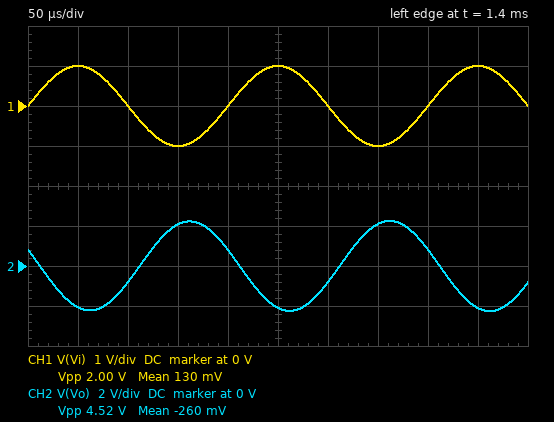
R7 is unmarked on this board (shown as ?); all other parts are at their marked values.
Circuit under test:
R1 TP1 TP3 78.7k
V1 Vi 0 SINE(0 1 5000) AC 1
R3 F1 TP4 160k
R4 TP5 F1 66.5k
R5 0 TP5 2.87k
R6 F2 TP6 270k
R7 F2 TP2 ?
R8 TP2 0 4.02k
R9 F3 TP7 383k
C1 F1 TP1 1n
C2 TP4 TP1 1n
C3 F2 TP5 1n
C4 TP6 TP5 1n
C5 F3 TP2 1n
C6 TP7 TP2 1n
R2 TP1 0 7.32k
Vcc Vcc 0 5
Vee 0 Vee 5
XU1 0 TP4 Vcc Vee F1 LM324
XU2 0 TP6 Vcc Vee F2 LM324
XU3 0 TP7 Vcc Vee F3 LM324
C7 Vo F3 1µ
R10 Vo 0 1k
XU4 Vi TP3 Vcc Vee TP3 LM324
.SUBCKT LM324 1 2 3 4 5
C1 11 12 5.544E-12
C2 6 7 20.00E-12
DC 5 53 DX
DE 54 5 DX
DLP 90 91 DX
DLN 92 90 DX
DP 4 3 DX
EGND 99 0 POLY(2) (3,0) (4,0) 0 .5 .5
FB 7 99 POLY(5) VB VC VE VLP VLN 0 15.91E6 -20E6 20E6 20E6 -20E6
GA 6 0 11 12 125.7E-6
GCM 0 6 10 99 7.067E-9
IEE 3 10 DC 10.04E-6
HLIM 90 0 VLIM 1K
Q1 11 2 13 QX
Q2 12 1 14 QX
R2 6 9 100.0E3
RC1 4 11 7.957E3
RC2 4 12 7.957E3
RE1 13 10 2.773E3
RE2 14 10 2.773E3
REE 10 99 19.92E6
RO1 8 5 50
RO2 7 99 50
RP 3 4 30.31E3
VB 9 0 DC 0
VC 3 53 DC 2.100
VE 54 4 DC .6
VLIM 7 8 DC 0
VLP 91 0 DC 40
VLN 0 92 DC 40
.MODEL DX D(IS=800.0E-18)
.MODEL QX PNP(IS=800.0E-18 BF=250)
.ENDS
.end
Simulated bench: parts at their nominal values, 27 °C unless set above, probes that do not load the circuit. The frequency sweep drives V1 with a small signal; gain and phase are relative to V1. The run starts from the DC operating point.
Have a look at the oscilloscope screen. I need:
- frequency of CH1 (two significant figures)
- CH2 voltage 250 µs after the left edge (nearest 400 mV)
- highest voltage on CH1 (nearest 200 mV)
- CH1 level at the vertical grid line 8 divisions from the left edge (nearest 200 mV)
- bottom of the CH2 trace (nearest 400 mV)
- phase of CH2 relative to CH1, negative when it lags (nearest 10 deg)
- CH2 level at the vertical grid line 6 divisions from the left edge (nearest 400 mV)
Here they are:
5.0 kHz
-2.0 V
1.0 V
0 V
-2.4 V
160 deg
-800 mV
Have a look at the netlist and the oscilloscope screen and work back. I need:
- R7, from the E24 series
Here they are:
47 kΩ
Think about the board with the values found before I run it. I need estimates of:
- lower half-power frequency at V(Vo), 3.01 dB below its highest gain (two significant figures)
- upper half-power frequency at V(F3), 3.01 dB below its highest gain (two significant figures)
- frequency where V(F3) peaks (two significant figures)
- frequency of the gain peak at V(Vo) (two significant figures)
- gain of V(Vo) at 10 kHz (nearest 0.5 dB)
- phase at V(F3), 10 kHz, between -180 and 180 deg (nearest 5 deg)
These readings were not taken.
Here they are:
4.0 kHz
5.8 kHz
4.5 kHz
4.5 kHz
-30.0 dB
-65 deg
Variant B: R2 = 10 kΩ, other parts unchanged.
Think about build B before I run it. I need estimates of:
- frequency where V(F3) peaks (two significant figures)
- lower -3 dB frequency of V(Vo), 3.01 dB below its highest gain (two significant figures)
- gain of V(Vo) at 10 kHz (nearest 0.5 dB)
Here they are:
4.3 kHz
3.9 kHz
-30.5 dB
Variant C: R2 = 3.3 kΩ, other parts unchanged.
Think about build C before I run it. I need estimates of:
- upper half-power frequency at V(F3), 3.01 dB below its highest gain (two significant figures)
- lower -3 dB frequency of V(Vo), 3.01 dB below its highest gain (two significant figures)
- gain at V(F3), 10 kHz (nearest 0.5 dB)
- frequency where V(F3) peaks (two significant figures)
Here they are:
6.4 kHz
5.1 kHz
-27.0 dB
5.7 kHz
